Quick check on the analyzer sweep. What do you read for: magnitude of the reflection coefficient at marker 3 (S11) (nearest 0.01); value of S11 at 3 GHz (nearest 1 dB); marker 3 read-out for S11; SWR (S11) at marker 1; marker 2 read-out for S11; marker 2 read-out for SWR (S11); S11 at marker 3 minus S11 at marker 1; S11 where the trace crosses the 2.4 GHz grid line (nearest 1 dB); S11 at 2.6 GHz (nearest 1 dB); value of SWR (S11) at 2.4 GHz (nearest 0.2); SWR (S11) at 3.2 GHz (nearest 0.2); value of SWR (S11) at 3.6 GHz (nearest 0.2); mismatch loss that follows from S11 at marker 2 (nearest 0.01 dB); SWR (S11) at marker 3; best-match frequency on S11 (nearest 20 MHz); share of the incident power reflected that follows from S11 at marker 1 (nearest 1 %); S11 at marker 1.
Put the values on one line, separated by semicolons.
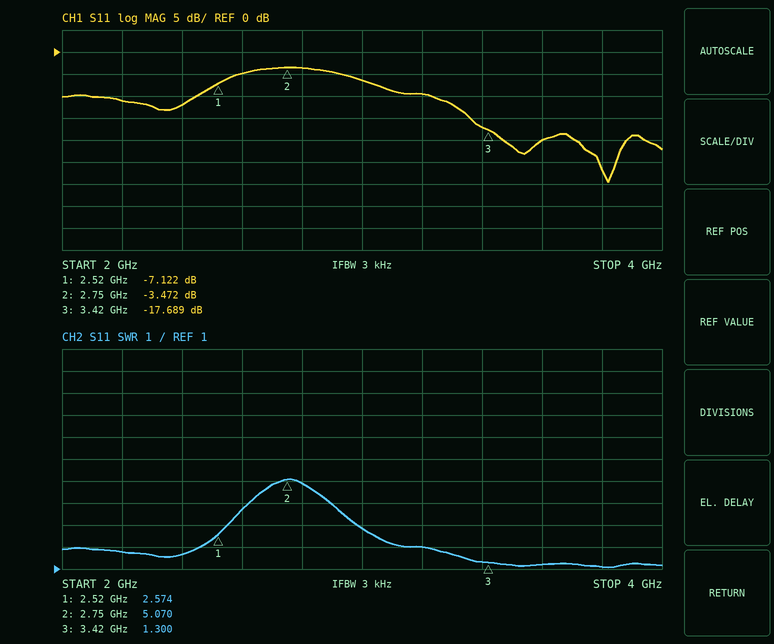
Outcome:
0.13; -6 dB; -17.689 dB; 2.574; -3.472 dB; 5.070; -10.567 dB; -12 dB; -5 dB; 1.6; 2.0; 1.2; 2.59 dB; 1.300; 3.82 GHz; 19 %; -7.122 dB
